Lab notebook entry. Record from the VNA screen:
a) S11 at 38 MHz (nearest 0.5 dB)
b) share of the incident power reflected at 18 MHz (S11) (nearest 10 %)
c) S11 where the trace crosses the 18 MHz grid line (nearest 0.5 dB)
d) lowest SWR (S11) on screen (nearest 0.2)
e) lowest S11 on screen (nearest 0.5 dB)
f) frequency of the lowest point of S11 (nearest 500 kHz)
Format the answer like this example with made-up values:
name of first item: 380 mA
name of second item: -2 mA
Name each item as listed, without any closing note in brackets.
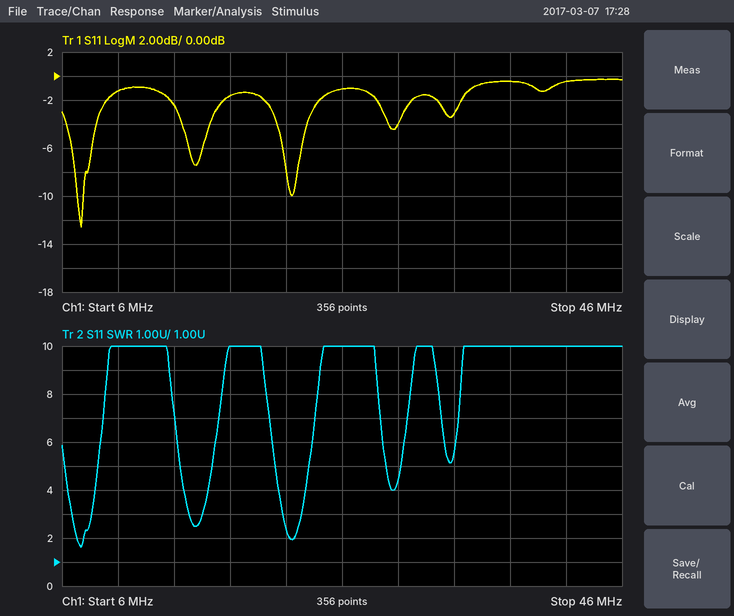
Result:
S11 at 38 MHz: -0.5 dB
share of the incident power reflected at 18 MHz (S11): 70 %
S11 where the trace crosses the 18 MHz grid line: -1.5 dB
lowest SWR (S11) on screen: 1.6
lowest S11 on screen: -12.5 dB
frequency of the lowest point of S11: 7.5 MHz
